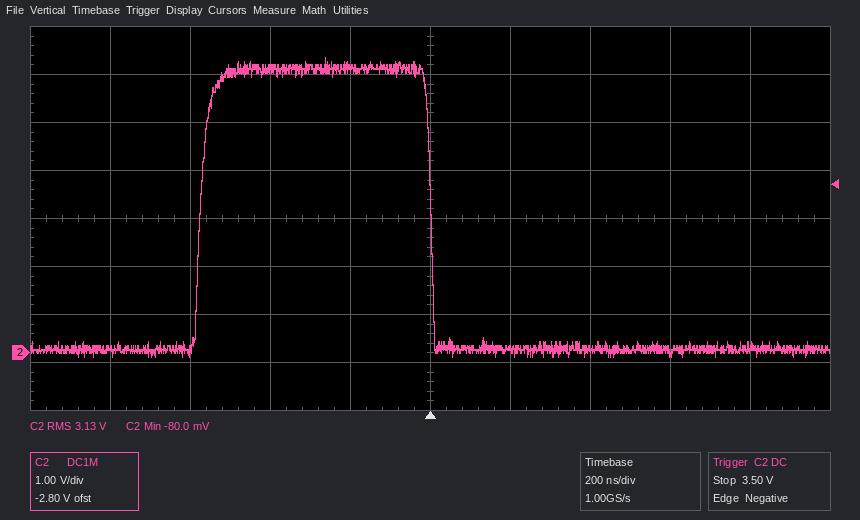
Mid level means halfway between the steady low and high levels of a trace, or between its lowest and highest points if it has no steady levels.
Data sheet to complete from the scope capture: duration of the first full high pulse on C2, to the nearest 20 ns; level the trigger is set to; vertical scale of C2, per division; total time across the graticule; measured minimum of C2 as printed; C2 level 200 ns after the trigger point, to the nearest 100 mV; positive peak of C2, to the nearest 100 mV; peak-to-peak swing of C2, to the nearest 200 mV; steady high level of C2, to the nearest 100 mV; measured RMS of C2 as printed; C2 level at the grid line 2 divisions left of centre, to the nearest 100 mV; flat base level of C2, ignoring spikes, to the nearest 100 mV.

580 ns
3.50 V
1 V
2 µs
-80.0 mV
100 mV
6.2 V
6.2 V
5.9 V
3.13 V
5.9 V
100 mV
